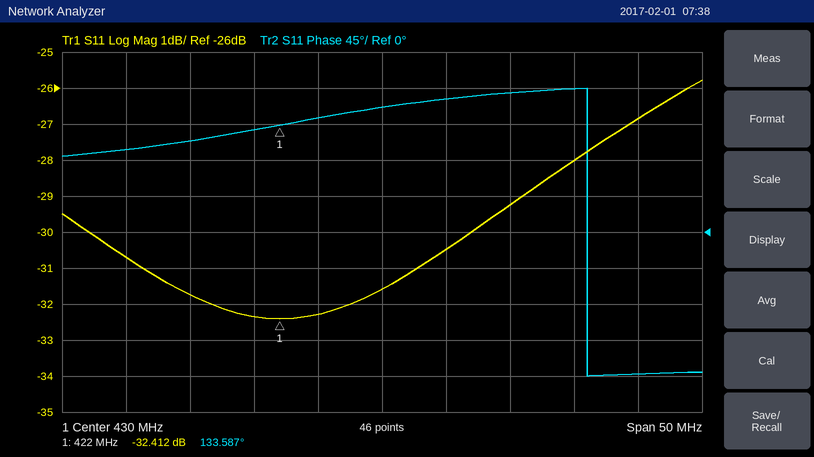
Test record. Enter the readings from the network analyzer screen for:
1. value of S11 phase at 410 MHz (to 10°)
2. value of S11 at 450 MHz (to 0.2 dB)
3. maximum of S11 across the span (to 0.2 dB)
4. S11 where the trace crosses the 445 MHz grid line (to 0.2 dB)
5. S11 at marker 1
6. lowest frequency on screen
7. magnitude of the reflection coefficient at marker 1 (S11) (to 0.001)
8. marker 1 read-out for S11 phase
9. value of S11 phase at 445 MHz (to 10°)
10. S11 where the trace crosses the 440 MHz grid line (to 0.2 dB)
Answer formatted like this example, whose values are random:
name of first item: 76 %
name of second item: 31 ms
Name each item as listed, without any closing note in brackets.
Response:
value of S11 phase at 410 MHz: 100°
value of S11 at 450 MHz: -26.8 dB
maximum of S11 across the span: -25.8 dB
S11 where the trace crosses the 445 MHz grid line: -28.0 dB
S11 at marker 1: -32.412 dB
lowest frequency on screen: 405 MHz
magnitude of the reflection coefficient at marker 1 (S11): 0.024
marker 1 read-out for S11 phase: 133.587°
value of S11 phase at 445 MHz: 180°
S11 where the trace crosses the 440 MHz grid line: -29.2 dB
